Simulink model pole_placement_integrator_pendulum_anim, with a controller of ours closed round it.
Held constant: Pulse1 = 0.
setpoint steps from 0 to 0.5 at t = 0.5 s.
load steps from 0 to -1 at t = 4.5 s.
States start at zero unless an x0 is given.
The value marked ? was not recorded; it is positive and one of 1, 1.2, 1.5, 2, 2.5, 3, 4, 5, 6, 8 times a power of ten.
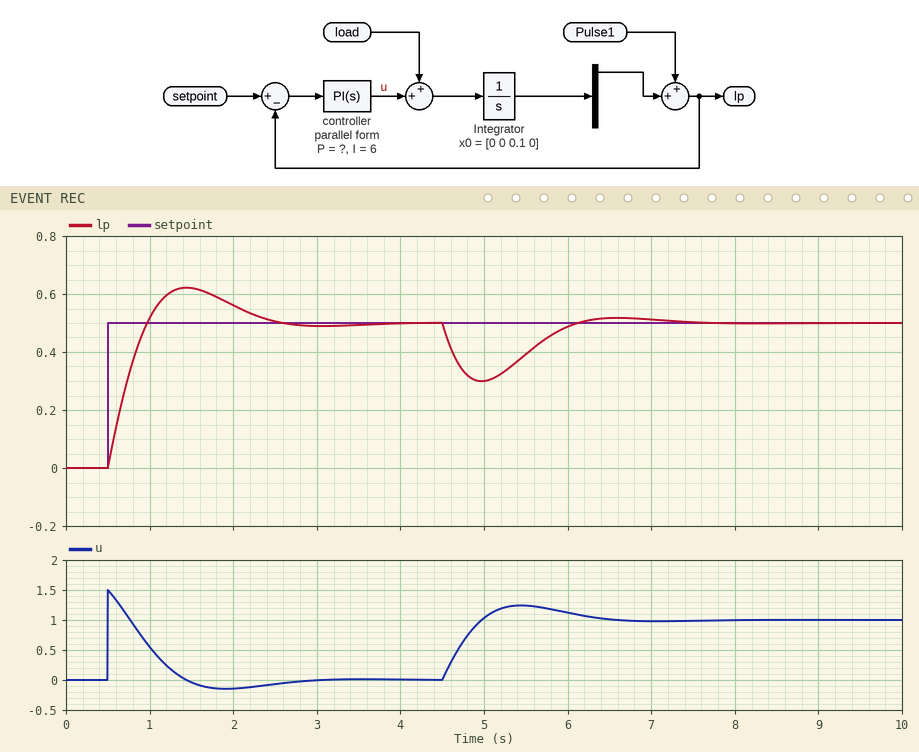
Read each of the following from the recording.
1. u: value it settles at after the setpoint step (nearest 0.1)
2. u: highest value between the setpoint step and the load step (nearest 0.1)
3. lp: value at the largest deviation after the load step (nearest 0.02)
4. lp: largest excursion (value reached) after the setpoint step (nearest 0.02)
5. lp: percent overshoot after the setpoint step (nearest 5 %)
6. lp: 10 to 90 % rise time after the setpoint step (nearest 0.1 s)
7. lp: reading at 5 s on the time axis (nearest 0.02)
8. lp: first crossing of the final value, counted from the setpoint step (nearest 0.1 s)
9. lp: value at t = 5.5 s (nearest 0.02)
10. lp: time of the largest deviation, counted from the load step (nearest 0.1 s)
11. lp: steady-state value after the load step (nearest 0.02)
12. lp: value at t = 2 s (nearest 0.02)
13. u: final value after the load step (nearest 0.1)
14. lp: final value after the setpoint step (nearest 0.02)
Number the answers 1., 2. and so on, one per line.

1. 0.0
2. 1.5
3. 0.30
4. 0.62
5. 25 %
6. 0.4 s
7. 0.30
8. 0.5 s
9. 0.40
10. 0.5 s
11. 0.50
12. 0.56
13. 1.0
14. 0.50
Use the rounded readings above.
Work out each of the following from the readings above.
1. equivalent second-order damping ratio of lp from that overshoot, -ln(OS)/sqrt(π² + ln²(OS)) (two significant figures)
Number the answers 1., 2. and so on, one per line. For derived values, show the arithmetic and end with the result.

1. ln(0.25) = -1.386; 1.386 / sqrt(9.870 + 1.922) = 0.40
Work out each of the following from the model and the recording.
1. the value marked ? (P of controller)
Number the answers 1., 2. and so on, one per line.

1. 3
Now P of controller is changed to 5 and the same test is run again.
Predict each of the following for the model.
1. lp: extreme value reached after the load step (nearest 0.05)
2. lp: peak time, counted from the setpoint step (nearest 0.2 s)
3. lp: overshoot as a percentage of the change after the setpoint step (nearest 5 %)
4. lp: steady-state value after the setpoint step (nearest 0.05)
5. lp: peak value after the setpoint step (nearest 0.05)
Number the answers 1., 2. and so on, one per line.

1. 0.35
2. 0.8 s
3. 15 %
4. 0.50
5. 0.55
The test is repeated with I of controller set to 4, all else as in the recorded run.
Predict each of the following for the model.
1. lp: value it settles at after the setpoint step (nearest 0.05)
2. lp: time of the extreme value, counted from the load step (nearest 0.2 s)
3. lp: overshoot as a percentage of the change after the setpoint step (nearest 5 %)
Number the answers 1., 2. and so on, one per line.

1. 0.50
2. 0.6 s
3. 20 %
